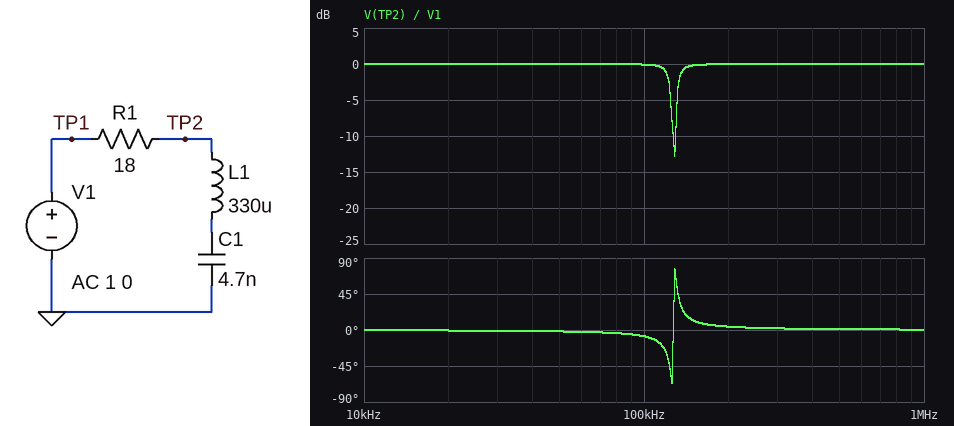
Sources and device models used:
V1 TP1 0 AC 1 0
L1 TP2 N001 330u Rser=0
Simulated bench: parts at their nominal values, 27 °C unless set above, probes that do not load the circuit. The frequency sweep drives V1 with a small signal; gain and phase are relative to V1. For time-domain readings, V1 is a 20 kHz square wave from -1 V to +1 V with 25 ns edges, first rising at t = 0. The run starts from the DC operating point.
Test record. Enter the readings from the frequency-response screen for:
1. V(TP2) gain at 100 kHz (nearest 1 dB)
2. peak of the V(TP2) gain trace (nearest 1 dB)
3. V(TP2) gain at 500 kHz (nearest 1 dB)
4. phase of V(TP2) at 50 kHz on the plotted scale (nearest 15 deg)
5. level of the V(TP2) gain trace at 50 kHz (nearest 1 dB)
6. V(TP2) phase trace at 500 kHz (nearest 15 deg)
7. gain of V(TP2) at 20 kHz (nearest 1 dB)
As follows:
0 dB
0 dB
0 dB
0 deg
0 dB
0 deg
0 dB
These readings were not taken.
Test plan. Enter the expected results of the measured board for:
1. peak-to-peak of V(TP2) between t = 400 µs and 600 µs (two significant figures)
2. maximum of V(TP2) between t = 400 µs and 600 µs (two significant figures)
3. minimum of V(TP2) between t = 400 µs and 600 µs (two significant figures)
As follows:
2.2 V
1.1 V
-1.1 V
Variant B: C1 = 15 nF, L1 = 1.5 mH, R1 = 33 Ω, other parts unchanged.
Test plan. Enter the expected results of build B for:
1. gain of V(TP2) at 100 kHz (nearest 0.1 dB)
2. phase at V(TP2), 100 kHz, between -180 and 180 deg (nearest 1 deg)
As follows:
0 dB
2 deg
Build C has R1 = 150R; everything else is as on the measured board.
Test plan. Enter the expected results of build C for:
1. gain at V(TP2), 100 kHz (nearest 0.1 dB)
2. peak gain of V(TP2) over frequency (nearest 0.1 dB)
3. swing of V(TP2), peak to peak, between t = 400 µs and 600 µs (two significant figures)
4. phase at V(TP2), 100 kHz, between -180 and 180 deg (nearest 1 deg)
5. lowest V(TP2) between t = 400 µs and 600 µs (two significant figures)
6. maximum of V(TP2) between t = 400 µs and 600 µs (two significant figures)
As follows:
-3.6 dB
0 dB
2.6 V
-49 deg
-1.3 V
1.3 V
